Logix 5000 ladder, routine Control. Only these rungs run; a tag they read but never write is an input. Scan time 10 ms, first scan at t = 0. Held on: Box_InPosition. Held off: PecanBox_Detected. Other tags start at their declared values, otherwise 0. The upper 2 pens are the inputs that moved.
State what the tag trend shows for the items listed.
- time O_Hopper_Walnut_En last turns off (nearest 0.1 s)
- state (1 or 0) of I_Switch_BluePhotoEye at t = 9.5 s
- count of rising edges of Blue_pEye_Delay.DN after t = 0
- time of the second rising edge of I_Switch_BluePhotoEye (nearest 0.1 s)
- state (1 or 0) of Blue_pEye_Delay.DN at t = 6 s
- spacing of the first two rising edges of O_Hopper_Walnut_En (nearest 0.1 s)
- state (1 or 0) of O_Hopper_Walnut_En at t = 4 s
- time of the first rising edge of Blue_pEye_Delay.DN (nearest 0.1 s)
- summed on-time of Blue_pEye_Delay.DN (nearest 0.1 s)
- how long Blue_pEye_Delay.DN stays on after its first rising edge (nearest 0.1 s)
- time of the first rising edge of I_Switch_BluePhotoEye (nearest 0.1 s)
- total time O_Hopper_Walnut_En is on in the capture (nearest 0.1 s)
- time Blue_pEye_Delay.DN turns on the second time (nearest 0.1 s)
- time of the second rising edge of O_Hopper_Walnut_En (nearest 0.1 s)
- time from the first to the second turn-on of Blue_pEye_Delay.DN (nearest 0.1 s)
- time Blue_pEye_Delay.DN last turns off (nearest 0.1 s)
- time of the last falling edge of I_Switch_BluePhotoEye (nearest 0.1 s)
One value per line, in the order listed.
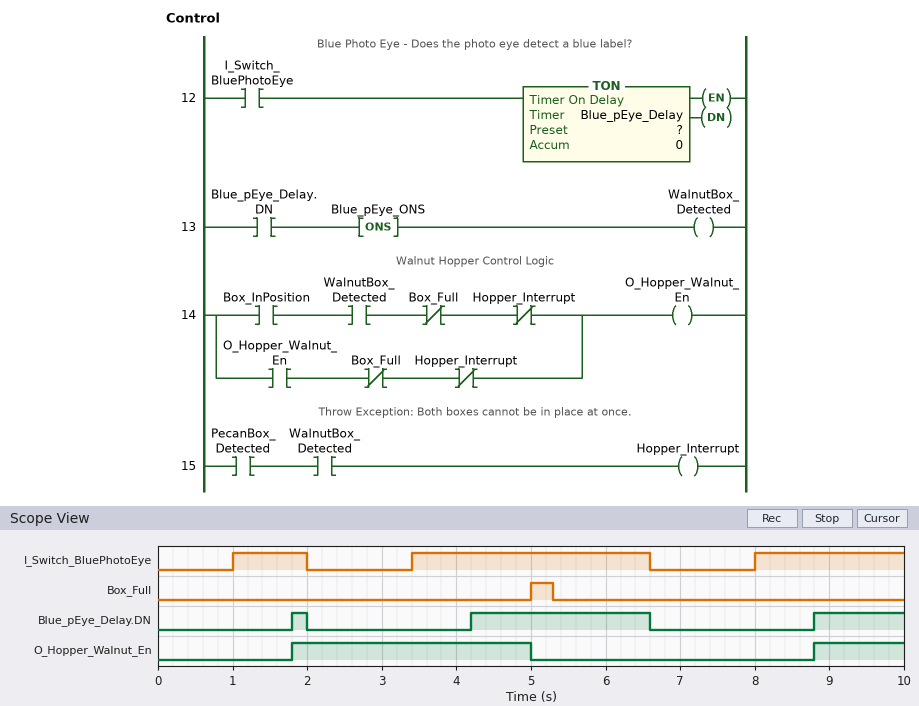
5.0 s
1
3
3.4 s
1
7.0 s
1
1.8 s
3.8 s
0.2 s
1.0 s
4.4 s
4.2 s
8.8 s
2.4 s
6.6 s
6.6 s
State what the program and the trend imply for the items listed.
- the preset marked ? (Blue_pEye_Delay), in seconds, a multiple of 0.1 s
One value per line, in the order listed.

0.8 s
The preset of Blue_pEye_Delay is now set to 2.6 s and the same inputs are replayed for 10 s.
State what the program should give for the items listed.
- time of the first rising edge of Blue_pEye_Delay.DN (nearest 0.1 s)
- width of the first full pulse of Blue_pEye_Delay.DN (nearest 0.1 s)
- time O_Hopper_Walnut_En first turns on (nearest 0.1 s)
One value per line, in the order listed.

6.0 s
0.6 s
6.0 s
